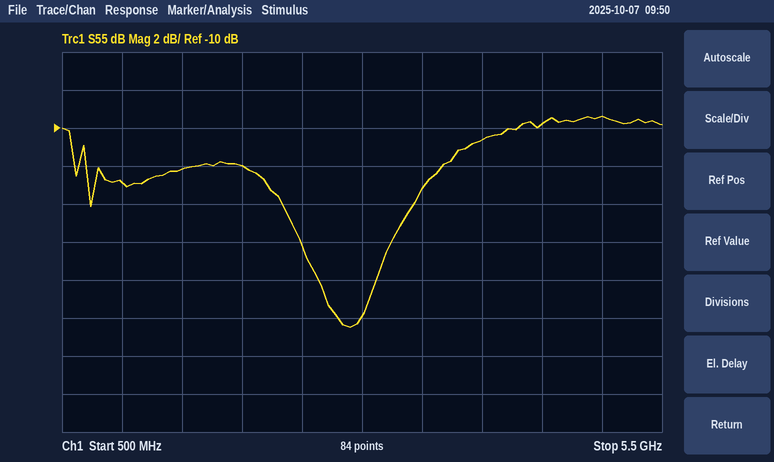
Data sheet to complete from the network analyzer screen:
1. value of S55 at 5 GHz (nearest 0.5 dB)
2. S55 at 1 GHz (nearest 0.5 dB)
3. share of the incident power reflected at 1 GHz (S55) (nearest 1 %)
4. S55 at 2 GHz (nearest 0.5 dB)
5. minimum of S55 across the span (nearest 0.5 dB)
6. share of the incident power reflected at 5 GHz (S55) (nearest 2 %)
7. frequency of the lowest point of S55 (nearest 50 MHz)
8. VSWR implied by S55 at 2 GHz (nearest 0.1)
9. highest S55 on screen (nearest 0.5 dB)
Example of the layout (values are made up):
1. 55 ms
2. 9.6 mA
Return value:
1. -9.5 dB
2. -13.0 dB
3. 5 %
4. -12.0 dB
5. -20.5 dB
6. 12 %
7. 2.90 GHz
8. 1.7
9. -9.5 dB
